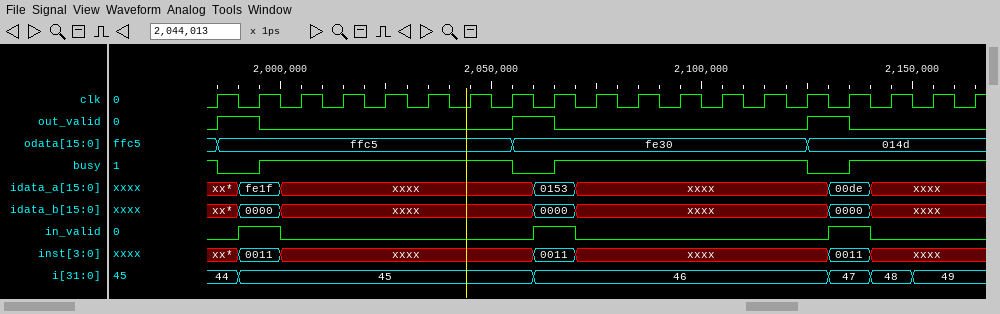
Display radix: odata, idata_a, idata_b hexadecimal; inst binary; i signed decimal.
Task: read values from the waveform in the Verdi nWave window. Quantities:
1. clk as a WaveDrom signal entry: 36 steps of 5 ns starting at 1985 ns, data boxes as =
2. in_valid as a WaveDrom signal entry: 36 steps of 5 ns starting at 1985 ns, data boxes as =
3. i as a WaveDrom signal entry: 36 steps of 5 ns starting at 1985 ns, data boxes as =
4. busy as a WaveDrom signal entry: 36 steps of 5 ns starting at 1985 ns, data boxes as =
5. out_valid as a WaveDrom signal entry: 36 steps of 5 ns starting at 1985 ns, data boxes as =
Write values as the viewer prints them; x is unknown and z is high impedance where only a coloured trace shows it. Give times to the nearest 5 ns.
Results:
{name: 'clk', wave: '101010101010101010101010101010101010'}
{name: 'in_valid', wave: '01.0...........1.0...........1.0....'}
{name: 'i', wave: '==.............=.............=.=.=..', data: '44 45 46 47 48 49'}
{name: 'busy', wave: '0.1...........0.1...........0.1.....'}
{name: 'out_valid', wave: '1.0...........1.0...........1.0.....'}
